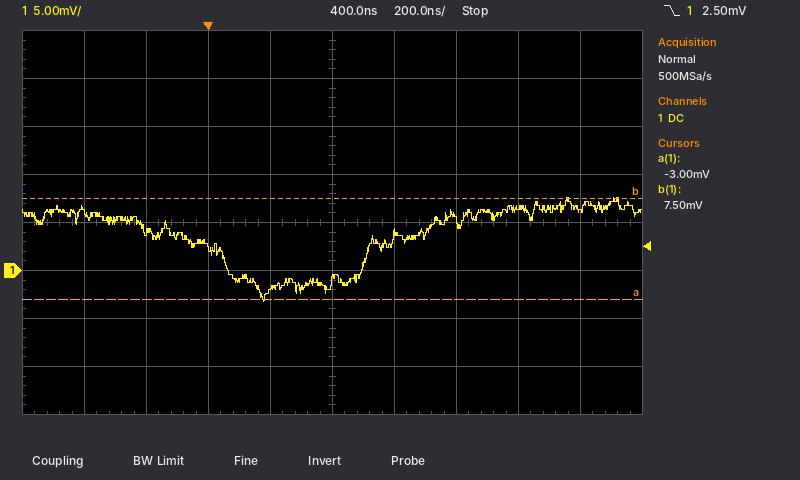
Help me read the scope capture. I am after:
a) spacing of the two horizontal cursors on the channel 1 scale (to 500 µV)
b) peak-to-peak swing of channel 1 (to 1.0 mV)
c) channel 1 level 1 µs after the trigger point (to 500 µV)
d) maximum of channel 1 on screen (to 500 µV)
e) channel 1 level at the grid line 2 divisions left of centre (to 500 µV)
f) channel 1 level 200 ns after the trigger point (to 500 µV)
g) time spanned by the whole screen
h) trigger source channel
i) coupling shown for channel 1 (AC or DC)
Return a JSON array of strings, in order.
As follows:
["10.5 mV", "11.0 mV", "6.5 mV", "7.5 mV", "2.5 mV", "-2.0 mV", "2 µs", "channel 1", "DC"]
